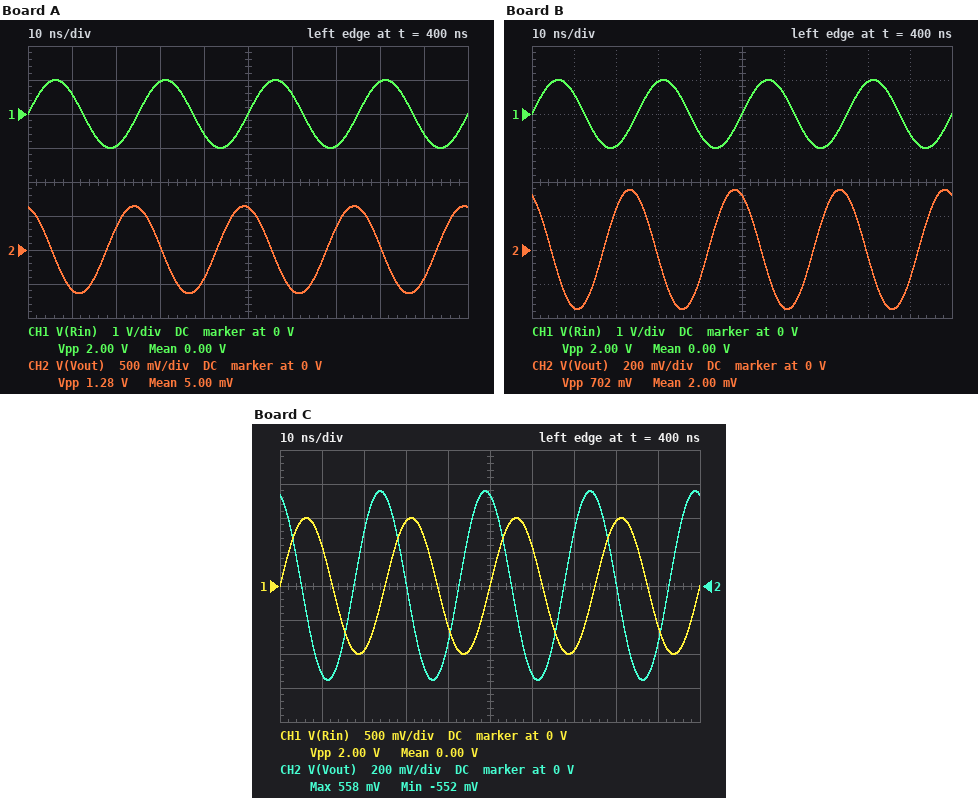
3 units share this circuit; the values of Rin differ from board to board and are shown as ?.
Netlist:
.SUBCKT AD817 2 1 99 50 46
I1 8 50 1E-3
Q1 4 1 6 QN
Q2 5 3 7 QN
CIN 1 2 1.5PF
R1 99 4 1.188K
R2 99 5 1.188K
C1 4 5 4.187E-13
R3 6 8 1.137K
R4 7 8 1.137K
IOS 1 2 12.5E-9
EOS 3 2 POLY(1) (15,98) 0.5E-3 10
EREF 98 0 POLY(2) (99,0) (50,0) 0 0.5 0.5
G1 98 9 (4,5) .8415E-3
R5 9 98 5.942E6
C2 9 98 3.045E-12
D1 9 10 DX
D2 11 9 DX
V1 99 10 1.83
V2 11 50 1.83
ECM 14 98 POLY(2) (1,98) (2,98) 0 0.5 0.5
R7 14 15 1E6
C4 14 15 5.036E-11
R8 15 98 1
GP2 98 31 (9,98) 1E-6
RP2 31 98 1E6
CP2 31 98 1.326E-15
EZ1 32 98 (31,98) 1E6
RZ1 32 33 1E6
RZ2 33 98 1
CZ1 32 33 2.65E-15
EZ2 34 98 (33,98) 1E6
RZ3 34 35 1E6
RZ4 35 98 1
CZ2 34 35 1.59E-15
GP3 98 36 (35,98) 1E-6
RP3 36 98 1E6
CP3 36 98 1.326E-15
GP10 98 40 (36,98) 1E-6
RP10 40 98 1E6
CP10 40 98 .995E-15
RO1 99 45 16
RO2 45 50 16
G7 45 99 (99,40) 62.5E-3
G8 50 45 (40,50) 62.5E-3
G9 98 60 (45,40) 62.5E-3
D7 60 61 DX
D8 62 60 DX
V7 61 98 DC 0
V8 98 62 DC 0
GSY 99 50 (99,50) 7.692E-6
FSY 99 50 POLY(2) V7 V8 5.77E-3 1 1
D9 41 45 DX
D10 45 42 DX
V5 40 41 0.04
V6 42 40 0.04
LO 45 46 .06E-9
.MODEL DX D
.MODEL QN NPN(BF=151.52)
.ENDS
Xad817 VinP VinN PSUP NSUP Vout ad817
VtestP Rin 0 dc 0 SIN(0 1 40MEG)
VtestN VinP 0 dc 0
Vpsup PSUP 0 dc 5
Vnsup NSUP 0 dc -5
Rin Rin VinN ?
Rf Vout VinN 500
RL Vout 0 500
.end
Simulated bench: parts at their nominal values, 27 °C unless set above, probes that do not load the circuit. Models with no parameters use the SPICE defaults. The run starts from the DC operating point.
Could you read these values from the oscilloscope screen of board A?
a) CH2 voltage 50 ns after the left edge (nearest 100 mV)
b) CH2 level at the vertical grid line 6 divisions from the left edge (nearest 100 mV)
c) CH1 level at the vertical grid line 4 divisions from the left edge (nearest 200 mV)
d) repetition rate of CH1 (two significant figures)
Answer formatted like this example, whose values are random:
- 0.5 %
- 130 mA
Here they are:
- 600 mV
- -600 mV
- -600 mV
- 40 MHz
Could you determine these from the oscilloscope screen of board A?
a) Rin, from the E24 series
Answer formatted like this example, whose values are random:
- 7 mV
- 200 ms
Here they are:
- 430 Ω
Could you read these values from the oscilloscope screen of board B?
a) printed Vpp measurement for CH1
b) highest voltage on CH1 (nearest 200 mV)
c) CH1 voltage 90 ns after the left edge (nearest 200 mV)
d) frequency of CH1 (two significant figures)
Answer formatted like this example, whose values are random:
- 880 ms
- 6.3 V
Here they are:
- 2.00 V
- 1.0 V
- -600 mV
- 40 MHz
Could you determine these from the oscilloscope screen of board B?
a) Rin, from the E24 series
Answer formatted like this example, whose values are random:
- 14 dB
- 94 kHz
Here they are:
- 1.1 kΩ
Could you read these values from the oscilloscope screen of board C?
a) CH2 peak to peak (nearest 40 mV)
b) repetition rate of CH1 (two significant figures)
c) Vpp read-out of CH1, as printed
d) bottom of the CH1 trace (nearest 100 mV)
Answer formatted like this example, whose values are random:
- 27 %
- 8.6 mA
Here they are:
- 1.12 V
- 40 MHz
- 2.00 V
- -1.0 V
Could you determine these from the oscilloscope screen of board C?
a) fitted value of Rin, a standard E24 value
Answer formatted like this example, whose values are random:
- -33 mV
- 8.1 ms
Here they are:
- 560 Ω
